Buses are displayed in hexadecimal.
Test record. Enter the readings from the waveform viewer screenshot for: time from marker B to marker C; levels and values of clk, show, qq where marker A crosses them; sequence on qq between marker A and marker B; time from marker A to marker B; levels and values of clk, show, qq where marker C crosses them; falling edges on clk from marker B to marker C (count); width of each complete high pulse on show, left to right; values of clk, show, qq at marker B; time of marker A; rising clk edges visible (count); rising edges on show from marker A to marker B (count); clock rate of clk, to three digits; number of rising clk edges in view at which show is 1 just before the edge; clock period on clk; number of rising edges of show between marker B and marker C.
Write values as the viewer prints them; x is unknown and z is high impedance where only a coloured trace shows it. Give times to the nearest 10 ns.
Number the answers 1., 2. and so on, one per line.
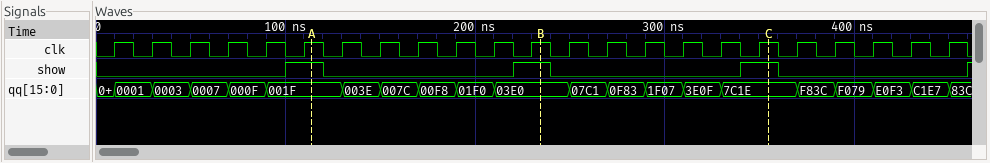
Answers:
1. 120 ns
2. clk=1, show=1, qq=001F
3. 001F, 003E, 007C, 00F8, 01F0, 03E0
4. 120 ns
5. clk=1, show=1, qq=7C1E
6. 6
7. 20 ns, 20 ns, 20 ns
8. clk=1, show=1, qq=03E0
9. 110 ns
10. 23
11. 1
12. 50.0 MHz
13. 3
14. 20 ns
15. 1
